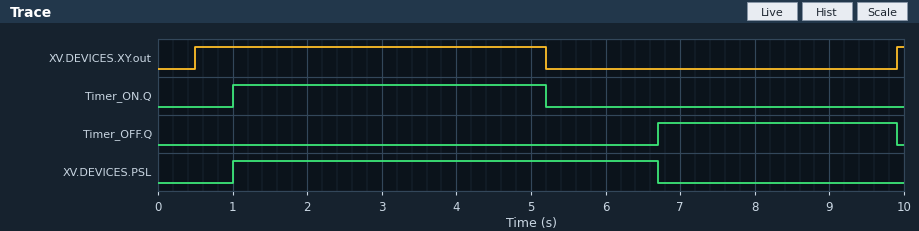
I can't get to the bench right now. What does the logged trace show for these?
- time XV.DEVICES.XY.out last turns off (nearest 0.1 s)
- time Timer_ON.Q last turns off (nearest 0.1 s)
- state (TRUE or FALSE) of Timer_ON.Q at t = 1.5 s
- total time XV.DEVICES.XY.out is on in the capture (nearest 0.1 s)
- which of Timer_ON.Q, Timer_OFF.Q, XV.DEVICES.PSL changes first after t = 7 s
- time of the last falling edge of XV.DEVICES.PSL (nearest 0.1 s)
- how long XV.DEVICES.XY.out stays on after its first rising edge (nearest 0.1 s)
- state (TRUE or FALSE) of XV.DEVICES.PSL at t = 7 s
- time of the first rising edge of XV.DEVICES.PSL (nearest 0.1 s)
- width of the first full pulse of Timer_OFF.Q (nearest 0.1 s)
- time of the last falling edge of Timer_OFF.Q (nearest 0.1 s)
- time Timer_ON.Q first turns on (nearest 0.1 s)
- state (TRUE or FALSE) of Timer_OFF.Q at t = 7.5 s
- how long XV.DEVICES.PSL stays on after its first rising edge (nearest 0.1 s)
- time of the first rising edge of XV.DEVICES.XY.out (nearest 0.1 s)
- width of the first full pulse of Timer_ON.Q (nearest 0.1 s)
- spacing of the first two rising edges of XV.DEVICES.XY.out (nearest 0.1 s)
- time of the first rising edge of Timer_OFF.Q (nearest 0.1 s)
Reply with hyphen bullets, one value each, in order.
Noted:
- 5.2 s
- 5.2 s
- TRUE
- 4.8 s
- Timer_OFF.Q
- 6.7 s
- 4.7 s
- FALSE
- 1.0 s
- 3.2 s
- 9.9 s
- 1.0 s
- TRUE
- 5.7 s
- 0.5 s
- 4.2 s
- 9.4 s
- 6.7 s
